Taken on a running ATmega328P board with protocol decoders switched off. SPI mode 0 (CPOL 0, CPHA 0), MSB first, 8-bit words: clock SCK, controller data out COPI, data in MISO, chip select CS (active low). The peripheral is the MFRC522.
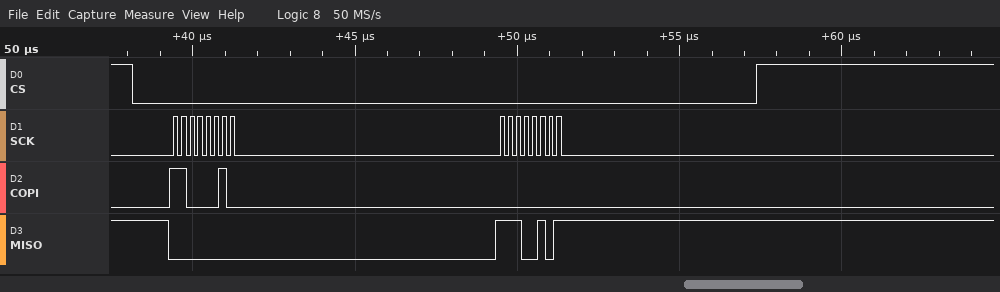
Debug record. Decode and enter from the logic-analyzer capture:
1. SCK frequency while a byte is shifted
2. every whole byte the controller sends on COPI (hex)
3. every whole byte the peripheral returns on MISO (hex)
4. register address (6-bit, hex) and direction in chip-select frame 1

4 MHz
C2 00
00 E5
0x21 read
